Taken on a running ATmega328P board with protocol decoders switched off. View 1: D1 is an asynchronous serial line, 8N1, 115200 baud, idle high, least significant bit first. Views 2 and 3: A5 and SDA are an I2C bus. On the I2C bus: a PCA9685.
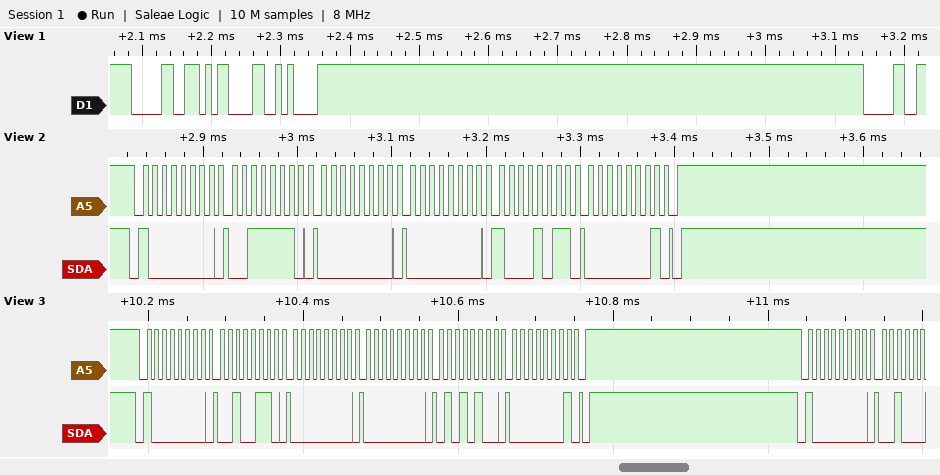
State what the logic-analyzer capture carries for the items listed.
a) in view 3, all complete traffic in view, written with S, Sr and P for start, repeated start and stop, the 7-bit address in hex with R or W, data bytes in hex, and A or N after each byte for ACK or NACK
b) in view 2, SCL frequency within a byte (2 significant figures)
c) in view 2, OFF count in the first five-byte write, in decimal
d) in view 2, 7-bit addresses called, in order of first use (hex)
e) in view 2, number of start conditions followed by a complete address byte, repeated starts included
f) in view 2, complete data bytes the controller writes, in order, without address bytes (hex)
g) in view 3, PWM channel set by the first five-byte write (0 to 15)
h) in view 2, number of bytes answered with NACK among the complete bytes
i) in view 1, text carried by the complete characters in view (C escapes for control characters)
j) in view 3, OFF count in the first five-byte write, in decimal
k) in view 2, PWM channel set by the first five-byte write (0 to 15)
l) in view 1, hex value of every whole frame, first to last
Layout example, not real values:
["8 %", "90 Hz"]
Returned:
["S 40W A 26 A 00 A 00 A 54 A 01 A P S 40W A", "100 kHz", "395", "0x40", "1", "3E 00 00 8B 01", "8", "0", "\"0\\r\\n0\"", "340", "14", "30 0D 0A 30"]
